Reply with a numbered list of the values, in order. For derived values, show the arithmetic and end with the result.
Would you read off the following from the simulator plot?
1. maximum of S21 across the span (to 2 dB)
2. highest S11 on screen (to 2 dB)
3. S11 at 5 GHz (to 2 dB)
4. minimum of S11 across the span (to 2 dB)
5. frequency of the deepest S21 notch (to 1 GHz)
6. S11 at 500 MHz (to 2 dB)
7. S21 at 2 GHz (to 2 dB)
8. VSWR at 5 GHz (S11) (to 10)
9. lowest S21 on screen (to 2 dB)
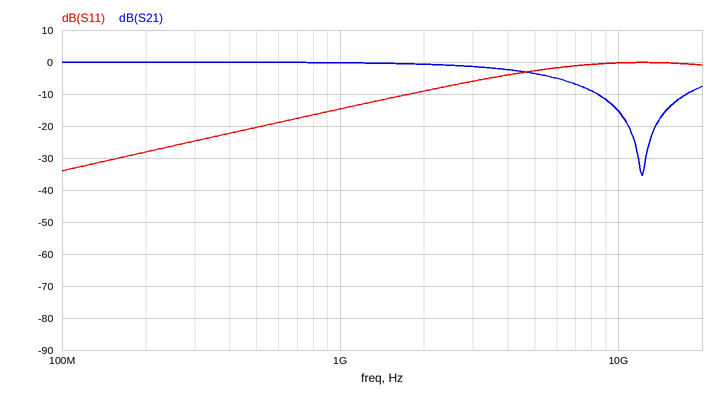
1. 0 dB
2. 0 dB
3. -2 dB
4. -34 dB
5. 12 GHz
6. -20 dB
7. 0 dB
8. |Γ| = 10^(-2/20) = 0.7943; VSWR = (1 + 0.7943)/(1 − 0.7943) ≈ 8.72, so 10 to the nearest 10
9. -36 dB
